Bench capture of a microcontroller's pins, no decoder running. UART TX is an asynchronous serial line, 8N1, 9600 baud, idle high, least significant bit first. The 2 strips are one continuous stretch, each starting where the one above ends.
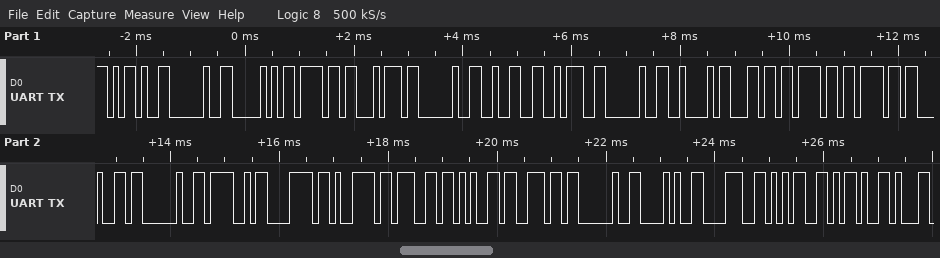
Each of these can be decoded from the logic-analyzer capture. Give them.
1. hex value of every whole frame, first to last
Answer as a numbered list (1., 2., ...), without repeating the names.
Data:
1. 0x2D 0x20 0x50 0x6F 0x74 0x20 0x32 0x3A 0x20 0x42 0x6C 0x6F 0x6F 0x64 0x20 0x4F 0x78 0x79 0x67 0x65 0x6E 0x20 0x28 0x38 0x35 0x2D
